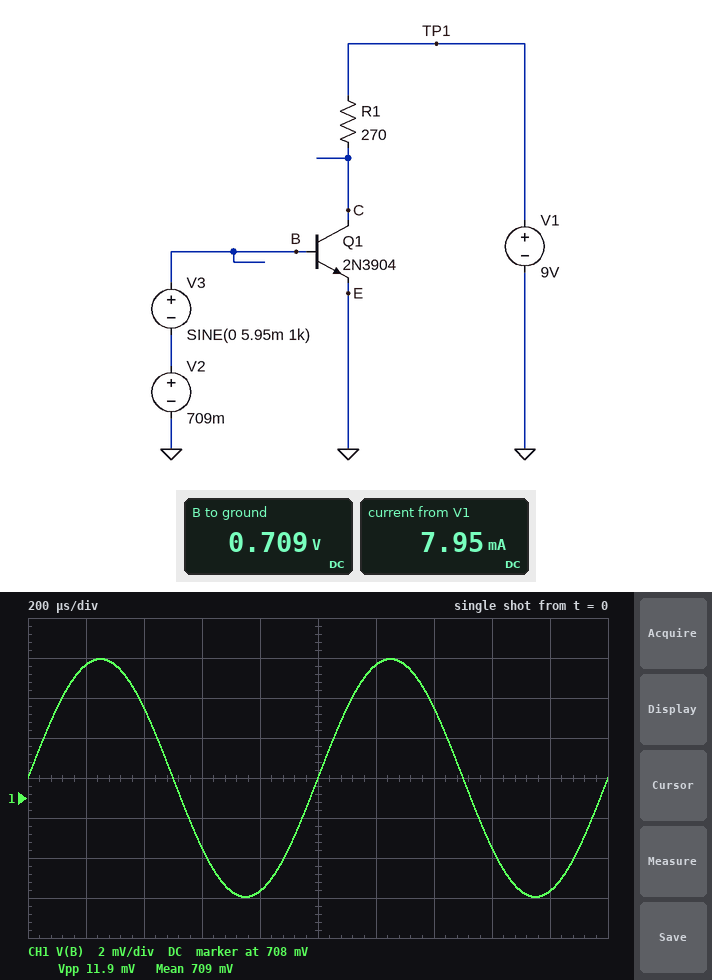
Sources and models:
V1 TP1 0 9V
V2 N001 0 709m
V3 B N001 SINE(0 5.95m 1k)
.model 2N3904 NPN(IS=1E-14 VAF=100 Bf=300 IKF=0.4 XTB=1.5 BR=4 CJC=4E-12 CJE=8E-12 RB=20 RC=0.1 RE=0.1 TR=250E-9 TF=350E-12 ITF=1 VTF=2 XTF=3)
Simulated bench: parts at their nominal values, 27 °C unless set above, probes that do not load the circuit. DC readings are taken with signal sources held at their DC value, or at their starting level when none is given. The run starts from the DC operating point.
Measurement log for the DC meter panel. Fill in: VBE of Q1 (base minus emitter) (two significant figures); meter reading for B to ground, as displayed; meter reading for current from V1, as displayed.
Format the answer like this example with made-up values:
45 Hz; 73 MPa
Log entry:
710 mV; 0.709 V; 7.95 mA
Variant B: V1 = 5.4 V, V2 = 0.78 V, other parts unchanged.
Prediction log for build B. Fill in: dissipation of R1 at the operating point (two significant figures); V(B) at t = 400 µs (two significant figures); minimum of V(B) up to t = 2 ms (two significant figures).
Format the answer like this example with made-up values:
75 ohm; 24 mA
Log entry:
110 mW; 780 mV; 770 mV
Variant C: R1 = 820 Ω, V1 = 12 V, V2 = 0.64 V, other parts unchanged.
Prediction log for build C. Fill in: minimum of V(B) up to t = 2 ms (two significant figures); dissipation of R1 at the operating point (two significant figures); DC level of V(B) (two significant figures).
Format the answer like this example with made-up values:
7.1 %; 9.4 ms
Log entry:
630 mV; 310 µW; 640 mV
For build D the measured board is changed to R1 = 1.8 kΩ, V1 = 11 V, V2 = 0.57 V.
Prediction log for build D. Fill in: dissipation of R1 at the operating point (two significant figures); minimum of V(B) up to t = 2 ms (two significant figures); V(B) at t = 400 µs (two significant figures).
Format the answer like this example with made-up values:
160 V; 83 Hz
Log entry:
3.0 µW; 560 mV; 570 mV
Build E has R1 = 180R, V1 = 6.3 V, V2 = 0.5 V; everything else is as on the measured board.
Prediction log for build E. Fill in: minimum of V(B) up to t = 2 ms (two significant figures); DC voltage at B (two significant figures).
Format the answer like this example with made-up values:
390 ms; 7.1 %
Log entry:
490 mV; 500 mV
